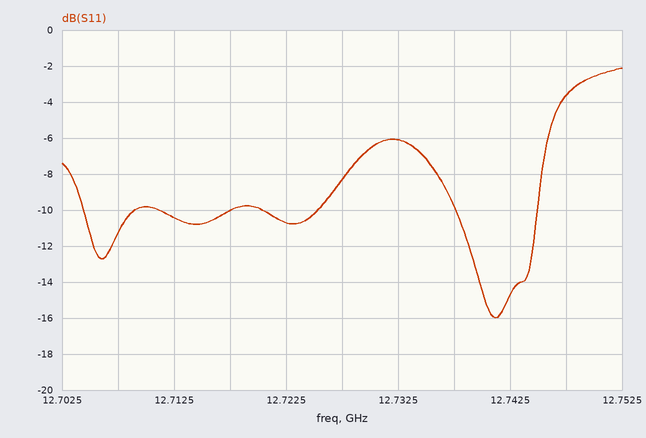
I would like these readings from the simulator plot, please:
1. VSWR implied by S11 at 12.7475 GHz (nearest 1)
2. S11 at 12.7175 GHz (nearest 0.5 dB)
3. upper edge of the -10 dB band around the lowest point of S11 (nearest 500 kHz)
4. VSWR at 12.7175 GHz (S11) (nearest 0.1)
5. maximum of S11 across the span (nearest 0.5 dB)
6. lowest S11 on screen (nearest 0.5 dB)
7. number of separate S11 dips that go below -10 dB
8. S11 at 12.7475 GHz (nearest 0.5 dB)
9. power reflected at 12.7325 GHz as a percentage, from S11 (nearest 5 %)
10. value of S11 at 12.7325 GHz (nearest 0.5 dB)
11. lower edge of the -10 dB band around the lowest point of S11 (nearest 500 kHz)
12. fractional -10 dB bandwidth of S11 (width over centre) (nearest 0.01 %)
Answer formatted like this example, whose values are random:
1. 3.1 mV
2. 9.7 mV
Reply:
1. 5
2. -10.0 dB
3. 12.7450 GHz
4. 1.9
5. -2.0 dB
6. -16.0 dB
7. 2
8. -3.5 dB
9. 25 %
10. -6.0 dB
11. 12.7375 GHz
12. 0.06 %
